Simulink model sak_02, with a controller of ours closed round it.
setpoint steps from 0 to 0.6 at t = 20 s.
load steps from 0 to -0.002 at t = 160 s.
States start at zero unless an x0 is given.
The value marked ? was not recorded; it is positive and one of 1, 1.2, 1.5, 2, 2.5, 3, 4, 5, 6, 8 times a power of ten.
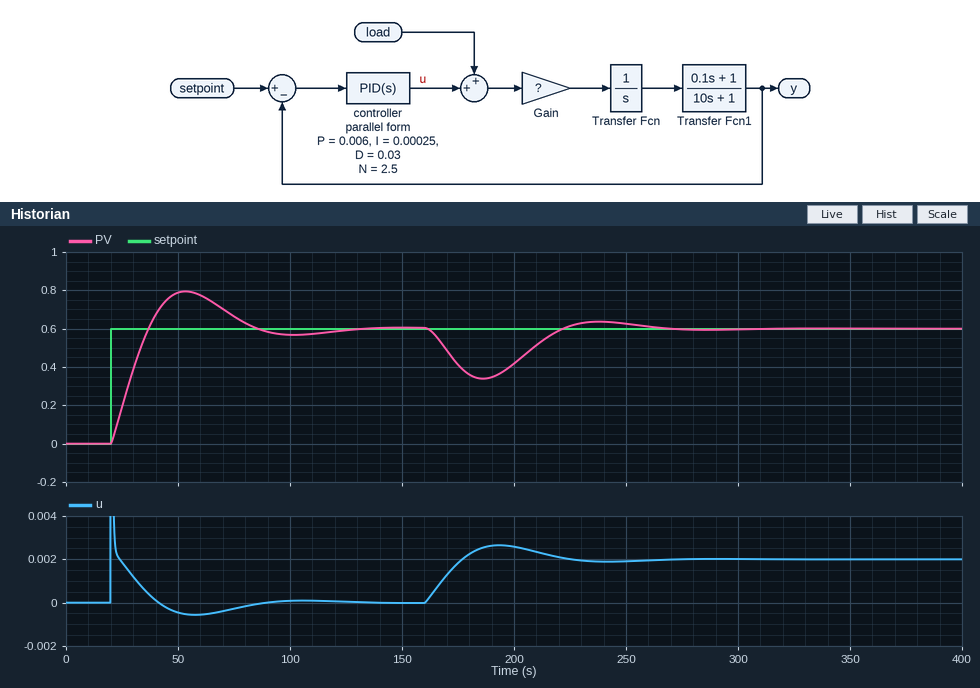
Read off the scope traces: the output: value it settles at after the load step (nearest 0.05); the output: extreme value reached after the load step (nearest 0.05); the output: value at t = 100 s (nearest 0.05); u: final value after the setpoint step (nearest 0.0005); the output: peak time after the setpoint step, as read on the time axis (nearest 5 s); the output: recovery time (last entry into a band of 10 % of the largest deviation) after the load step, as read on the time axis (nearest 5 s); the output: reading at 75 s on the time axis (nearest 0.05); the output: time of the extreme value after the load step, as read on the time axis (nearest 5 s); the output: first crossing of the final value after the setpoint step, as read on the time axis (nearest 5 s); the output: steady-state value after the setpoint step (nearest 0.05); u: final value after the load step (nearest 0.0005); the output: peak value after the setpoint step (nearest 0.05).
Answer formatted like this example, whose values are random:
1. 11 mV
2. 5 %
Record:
1. 0.60
2. 0.35
3. 0.55
4. 0.0000
5. 55 s
6. 250 s
7. 0.65
8. 185 s
9. 35 s
10. 0.60
11. 0.0020
12. 0.80
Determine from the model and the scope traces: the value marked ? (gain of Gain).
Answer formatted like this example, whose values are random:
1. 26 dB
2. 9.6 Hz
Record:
1. 20
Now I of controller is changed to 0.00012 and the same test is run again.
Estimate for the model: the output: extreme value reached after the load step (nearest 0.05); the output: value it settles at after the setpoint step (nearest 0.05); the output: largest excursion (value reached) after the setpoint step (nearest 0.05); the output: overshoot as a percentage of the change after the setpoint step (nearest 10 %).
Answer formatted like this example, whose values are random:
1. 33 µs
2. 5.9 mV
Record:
1. 0.30
2. 0.60
3. 0.70
4. 20 %
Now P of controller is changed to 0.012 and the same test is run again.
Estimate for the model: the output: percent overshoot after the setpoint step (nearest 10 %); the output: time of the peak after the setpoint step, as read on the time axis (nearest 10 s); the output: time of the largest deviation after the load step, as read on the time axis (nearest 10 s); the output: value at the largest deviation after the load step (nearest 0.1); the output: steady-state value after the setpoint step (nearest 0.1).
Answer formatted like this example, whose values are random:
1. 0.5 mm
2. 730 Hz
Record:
1. 30 %
2. 40 s
3. 180 s
4. 0.4
5. 0.6
